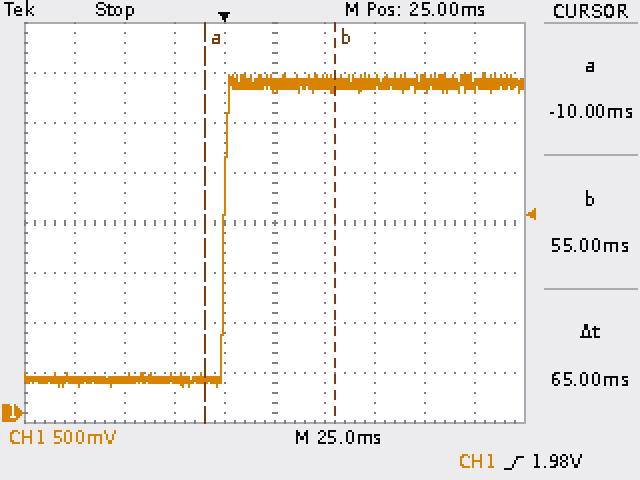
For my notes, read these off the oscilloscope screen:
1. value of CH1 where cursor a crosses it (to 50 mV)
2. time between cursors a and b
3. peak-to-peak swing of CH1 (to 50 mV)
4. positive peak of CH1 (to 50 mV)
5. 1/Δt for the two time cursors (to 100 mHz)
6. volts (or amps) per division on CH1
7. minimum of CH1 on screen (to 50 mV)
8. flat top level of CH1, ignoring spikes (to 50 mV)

350 mV
65 ms
3.15 V
3.40 V
15.4 Hz
500 mV
250 mV
3.30 V
